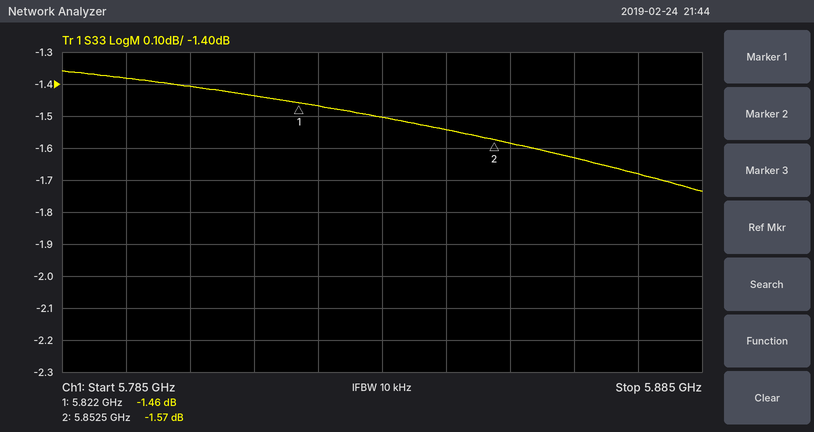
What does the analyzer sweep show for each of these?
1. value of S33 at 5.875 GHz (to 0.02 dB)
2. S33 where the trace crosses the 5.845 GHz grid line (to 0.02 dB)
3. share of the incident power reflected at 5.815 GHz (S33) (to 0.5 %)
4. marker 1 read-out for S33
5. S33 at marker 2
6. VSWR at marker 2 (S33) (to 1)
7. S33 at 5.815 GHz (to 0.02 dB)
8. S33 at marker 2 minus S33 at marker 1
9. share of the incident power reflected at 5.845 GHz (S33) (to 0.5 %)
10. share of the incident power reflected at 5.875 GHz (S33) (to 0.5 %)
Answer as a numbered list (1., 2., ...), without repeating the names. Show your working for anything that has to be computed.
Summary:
1. -1.68 dB
2. -1.54 dB
3. 10^(-1.44/10) ≈ 71.8 %, so 72.0 % to the nearest 0.5 %
4. -1.46 dB
5. -1.57 dB
6. (1 + 0.8346)/(1 − 0.8346) ≈ 11
7. -1.44 dB
8. -1.57 − (-1.46) = -0.11 dB
9. 10^(-1.54/10) ≈ 70.1 %, so 70.0 % to the nearest 0.5 %
10. 10^(-1.68/10) ≈ 67.9 %, so 68.0 % to the nearest 0.5 %
